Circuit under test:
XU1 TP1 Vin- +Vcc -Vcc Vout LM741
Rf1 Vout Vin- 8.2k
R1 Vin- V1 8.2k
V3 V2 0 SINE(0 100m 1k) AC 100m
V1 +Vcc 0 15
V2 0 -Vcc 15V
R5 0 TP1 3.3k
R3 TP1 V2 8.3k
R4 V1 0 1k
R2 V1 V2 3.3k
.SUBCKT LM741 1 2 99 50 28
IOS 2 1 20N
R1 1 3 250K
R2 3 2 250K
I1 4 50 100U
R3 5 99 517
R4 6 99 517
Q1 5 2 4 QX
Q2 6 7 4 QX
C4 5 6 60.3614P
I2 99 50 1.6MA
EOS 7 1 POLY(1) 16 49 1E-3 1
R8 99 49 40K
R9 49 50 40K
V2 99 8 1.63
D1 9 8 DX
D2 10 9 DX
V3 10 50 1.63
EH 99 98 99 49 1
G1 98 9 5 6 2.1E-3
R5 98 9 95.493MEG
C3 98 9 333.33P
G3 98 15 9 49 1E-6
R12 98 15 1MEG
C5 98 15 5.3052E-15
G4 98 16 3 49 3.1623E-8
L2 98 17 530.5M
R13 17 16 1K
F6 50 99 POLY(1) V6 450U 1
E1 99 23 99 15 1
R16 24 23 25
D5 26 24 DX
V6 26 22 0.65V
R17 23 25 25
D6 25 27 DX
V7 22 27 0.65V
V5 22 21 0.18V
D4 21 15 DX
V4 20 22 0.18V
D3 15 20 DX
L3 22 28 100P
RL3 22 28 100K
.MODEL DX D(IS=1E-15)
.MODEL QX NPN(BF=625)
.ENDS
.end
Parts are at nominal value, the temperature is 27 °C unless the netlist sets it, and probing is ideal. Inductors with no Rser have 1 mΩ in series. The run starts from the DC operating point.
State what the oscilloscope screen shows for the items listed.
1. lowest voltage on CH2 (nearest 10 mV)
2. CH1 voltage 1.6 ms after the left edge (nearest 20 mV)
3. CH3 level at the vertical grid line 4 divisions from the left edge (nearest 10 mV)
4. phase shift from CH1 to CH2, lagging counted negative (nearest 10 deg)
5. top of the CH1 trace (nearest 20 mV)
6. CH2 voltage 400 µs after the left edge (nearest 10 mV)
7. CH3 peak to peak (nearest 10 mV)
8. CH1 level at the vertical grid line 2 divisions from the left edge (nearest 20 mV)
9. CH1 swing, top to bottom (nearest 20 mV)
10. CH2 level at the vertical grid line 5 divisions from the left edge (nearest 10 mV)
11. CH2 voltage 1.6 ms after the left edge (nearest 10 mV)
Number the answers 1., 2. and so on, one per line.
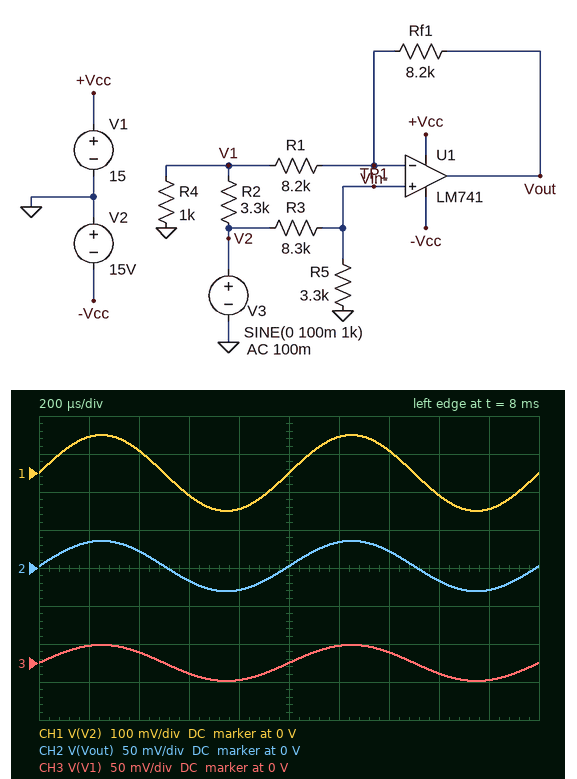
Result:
1. -30 mV
2. -60 mV
3. -20 mV
4. 0 deg
5. 100 mV
6. 20 mV
7. 50 mV
8. 60 mV
9. 200 mV
10. 0 V
11. -20 mV
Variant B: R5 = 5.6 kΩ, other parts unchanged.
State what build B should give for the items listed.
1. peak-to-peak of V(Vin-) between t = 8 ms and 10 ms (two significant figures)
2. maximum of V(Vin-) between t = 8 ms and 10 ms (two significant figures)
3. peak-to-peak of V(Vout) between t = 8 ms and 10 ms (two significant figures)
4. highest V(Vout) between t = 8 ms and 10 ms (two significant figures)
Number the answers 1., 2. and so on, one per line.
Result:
1. 81 mV
2. 41 mV
3. 110 mV
4. 58 mV
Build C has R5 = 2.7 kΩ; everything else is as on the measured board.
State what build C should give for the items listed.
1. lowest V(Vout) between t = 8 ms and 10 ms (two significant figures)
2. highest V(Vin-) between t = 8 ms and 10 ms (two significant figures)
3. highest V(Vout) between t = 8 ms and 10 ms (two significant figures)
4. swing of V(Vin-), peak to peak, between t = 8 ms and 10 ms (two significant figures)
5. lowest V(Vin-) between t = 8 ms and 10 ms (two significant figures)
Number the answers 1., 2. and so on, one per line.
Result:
1. -23 mV
2. 25 mV
3. 28 mV
4. 49 mV
5. -24 mV
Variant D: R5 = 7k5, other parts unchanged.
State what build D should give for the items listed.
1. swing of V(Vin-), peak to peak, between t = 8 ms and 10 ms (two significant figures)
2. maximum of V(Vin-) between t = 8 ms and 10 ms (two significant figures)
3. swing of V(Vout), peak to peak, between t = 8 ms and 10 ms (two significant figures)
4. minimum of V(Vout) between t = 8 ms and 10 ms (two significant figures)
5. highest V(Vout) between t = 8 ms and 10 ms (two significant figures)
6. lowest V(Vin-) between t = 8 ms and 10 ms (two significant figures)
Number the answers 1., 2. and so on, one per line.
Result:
1. 95 mV
2. 48 mV
3. 140 mV
4. -67 mV
5. 72 mV
6. -47 mV
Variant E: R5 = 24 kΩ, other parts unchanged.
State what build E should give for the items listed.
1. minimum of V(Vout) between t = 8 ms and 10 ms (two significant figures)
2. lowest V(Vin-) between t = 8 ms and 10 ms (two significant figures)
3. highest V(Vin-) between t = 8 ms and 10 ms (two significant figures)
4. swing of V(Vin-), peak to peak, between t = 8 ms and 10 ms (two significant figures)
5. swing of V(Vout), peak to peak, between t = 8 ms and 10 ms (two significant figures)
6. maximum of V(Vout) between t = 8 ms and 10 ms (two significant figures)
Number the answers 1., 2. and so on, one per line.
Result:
1. -120 mV
2. -74 mV
3. 75 mV
4. 150 mV
5. 240 mV
6. 120 mV
